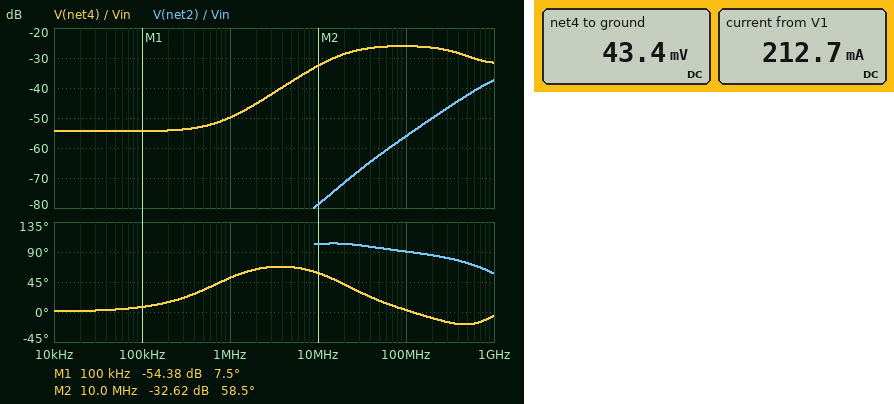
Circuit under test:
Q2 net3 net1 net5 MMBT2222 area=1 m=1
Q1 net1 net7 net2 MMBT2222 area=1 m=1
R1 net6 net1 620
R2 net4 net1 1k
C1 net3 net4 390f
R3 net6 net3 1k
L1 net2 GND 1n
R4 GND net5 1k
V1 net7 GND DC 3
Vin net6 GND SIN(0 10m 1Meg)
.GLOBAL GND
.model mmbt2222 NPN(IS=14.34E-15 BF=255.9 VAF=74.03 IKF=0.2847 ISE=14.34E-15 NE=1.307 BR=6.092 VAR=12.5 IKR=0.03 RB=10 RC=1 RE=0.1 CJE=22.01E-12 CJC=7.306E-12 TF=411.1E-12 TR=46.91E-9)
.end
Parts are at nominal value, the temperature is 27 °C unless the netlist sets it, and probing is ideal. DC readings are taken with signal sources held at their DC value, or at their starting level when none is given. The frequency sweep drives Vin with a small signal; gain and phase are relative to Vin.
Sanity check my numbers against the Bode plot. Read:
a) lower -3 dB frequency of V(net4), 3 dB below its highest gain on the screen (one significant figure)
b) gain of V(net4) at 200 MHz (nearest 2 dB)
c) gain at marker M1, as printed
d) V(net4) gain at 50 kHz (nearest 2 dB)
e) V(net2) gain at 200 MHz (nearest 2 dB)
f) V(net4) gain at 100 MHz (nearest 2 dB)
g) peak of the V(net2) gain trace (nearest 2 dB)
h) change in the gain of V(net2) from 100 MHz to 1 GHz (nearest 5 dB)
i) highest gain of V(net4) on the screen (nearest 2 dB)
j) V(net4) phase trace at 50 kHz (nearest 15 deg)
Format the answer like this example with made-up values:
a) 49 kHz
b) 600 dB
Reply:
a) 20 MHz
b) -26 dB
c) -54.38 dB
d) -54 dB
e) -50 dB
f) -26 dB
g) -38 dB
h) 20 dB
i) -26 dB
j) 0 deg
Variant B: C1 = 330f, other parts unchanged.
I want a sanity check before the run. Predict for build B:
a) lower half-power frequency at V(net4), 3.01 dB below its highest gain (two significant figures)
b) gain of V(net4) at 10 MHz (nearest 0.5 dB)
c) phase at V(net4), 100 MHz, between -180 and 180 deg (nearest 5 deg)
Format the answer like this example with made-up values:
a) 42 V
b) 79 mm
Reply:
a) 19 MHz
b) -34.0 dB
c) 5 deg
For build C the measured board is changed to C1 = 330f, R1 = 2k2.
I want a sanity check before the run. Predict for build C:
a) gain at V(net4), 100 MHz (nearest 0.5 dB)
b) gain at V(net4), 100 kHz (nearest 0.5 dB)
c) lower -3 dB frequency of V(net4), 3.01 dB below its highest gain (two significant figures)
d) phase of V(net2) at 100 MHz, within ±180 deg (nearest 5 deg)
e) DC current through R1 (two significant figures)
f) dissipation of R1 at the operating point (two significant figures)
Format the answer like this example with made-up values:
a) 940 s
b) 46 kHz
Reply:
a) -27.5 dB
b) -65.0 dB
c) 19 MHz
d) 95 deg
e) 20 µA
f) 860 nW
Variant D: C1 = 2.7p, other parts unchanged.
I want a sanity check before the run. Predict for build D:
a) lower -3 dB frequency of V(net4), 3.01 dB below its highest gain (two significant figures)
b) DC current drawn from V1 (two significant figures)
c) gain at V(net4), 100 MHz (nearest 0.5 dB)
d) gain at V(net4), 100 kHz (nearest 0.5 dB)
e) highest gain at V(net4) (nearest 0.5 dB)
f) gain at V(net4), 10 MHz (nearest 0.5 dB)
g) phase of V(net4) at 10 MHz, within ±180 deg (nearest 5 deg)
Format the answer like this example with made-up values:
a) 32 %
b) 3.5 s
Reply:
a) 11 MHz
b) 210 mA
c) -16.0 dB
d) -52.0 dB
e) -13.5 dB
f) -17.0 dB
g) 50 deg
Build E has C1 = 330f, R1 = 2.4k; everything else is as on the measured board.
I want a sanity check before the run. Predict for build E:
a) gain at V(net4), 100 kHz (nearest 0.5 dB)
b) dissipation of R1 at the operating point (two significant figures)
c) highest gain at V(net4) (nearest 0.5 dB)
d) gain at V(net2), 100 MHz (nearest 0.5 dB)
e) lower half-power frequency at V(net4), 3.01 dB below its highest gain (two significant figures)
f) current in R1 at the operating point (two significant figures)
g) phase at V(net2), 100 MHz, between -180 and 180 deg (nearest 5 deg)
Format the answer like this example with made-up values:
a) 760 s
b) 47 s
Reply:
a) -65.5 dB
b) 790 nW
c) -27.5 dB
d) -61.5 dB
e) 19 MHz
f) 18 µA
g) 95 deg
